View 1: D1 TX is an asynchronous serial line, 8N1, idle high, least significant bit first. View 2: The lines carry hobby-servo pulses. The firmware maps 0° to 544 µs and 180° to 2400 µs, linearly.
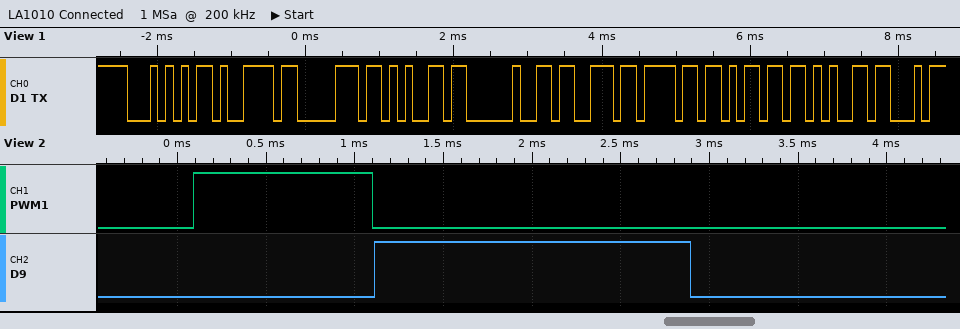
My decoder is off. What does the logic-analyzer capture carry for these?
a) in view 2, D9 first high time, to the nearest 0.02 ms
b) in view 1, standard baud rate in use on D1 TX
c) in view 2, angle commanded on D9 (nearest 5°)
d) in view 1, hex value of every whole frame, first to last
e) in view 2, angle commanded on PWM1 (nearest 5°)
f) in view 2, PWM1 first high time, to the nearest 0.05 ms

1.78 ms
9600 baud
120°
54 79 70 65 20 73 6F 6D 65
45°
1.00 ms
